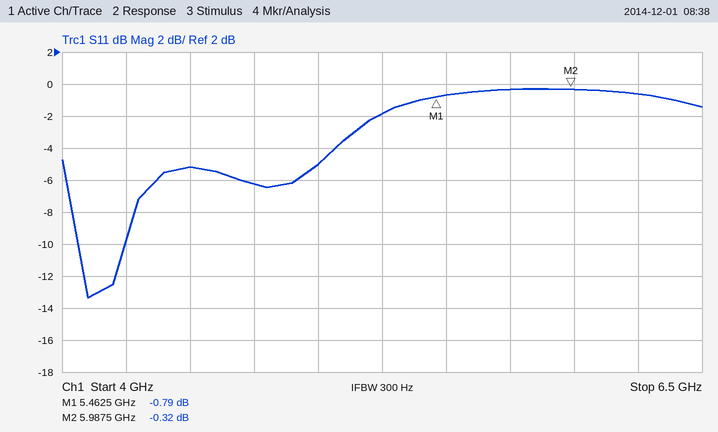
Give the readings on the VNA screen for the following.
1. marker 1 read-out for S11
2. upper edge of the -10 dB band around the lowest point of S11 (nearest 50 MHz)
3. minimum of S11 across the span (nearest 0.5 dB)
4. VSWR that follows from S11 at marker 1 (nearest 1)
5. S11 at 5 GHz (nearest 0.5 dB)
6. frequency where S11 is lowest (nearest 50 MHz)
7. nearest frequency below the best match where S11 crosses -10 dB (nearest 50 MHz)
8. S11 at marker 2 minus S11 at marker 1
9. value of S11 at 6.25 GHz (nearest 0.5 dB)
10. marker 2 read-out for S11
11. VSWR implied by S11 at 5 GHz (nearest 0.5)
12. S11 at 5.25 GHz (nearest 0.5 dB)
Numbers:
-0.79 dB
4.25 GHz
-13.5 dB
22
-5.0 dB
4.10 GHz
4.05 GHz
0.47 dB
-0.5 dB
-0.32 dB
3.5
-2.0 dB
